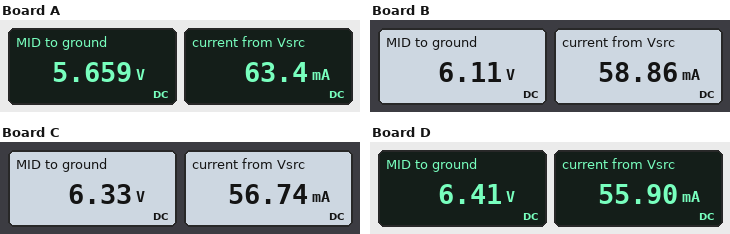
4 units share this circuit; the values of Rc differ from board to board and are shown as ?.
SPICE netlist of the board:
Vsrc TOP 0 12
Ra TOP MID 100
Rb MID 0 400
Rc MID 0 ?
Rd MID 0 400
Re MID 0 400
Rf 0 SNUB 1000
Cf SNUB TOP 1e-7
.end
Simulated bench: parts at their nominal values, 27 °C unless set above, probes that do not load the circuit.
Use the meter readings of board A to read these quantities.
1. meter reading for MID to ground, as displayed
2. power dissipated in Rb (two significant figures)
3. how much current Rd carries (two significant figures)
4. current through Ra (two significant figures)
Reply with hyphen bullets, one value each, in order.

- 5.659 V
- 80 mW
- 14 mA
- 63 mA
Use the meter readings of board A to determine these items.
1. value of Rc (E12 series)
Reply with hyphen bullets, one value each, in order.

- 270 Ω
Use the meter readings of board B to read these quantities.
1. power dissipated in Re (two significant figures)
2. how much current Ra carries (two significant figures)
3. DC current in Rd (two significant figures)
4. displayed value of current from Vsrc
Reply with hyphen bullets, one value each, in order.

- 93 mW
- 59 mA
- 15 mA
- 58.86 mA
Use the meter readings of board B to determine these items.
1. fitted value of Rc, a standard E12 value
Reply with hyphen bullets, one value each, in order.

- 470 Ω
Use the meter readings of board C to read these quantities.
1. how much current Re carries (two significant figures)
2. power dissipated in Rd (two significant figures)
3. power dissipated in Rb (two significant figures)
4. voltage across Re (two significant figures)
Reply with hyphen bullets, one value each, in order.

- 16 mA
- 100 mW
- 100 mW
- 6.3 V
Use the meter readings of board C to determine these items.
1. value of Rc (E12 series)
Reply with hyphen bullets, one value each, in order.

- 680 Ω
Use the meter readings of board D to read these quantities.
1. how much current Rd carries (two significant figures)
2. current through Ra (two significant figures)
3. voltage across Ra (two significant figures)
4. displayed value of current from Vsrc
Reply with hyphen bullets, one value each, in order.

- 16 mA
- 56 mA
- 5.6 V
- 55.90 mA
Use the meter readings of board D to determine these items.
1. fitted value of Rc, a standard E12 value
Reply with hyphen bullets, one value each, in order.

- 820 Ω
